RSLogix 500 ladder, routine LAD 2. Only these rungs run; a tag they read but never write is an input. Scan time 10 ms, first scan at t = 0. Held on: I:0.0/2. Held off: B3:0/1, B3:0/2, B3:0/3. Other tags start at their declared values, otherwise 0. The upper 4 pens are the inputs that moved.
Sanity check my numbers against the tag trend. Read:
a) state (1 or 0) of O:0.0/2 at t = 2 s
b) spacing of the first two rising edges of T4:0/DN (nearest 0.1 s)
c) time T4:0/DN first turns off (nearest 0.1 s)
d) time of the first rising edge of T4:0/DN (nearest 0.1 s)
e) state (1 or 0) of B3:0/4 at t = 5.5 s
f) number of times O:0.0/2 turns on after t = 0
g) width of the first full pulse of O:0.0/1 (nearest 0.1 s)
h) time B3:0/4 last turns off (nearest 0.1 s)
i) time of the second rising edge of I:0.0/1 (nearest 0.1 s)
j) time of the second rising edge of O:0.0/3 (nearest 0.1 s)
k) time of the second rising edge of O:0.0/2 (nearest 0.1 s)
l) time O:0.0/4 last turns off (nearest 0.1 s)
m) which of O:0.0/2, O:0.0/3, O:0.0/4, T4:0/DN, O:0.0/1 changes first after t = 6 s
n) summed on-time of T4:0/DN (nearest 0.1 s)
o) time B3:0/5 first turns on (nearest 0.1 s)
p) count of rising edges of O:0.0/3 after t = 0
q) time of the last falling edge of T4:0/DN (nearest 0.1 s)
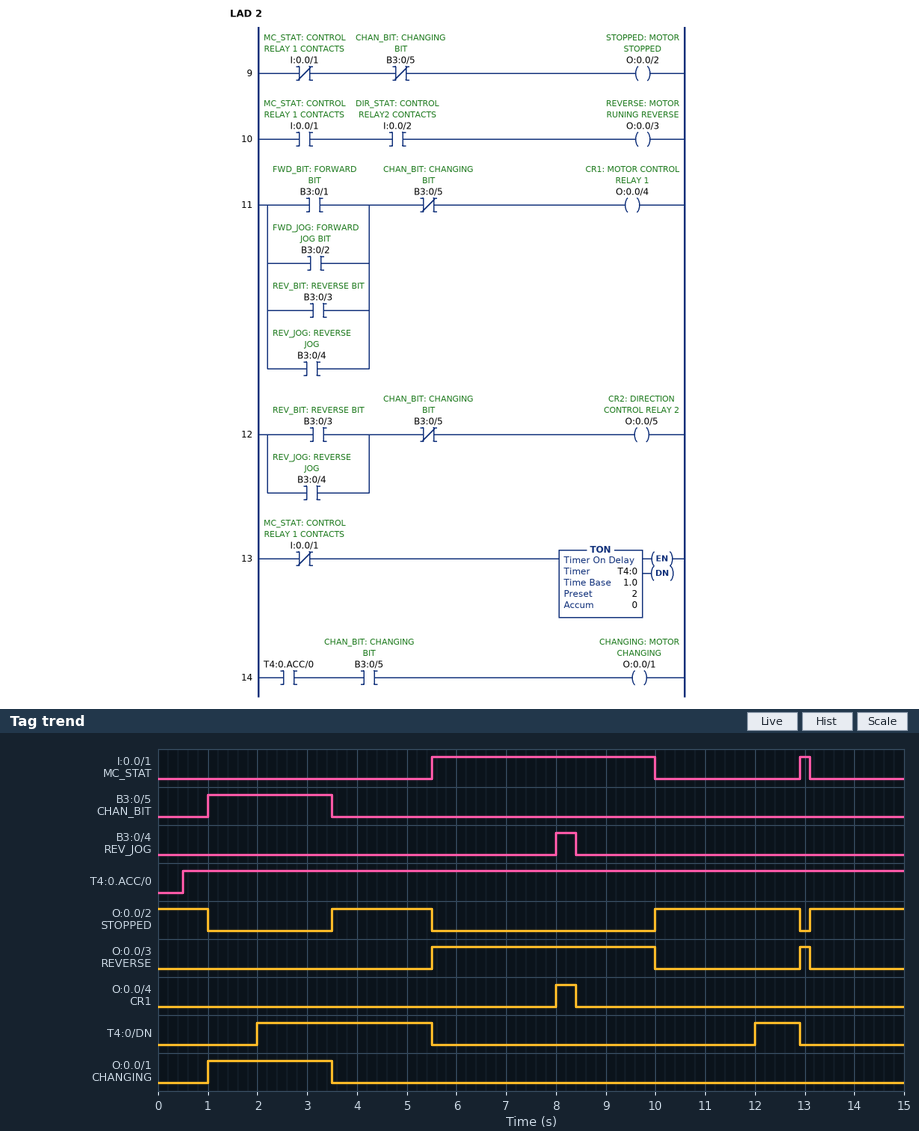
0
10.0 s
5.5 s
2.0 s
0
3
2.5 s
8.4 s
12.9 s
12.9 s
10.0 s
8.4 s
O:0.0/4
4.4 s
1.0 s
2
12.9 s
